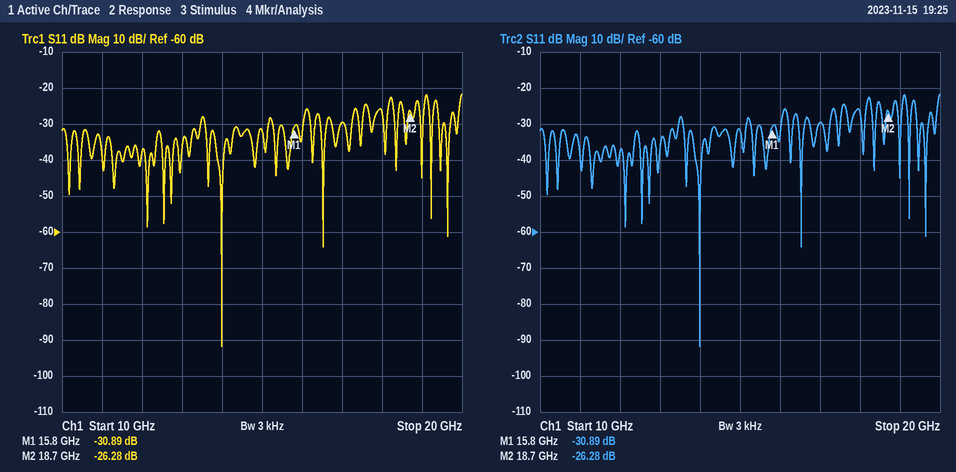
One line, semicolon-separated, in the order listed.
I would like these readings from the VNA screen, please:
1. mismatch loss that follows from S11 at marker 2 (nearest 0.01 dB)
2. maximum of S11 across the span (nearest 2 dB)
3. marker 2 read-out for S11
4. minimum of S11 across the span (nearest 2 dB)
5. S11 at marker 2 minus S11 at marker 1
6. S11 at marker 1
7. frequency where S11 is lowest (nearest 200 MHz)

0.01 dB; -22 dB; -26.28 dB; -92 dB; 4.61 dB; -30.89 dB; 14.0 GHz
